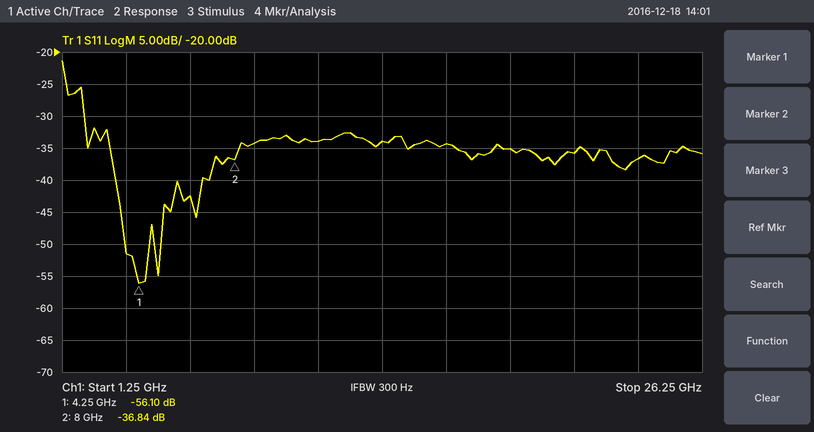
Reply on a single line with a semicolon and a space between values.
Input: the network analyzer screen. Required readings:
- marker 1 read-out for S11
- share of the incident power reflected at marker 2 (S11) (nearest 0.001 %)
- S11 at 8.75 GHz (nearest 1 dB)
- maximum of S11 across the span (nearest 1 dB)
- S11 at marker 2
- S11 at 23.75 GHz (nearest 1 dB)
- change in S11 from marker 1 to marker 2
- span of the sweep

-56.10 dB; 0.021 %; -34 dB; -21 dB; -36.84 dB; -37 dB; 19.26 dB; 25 GHz
